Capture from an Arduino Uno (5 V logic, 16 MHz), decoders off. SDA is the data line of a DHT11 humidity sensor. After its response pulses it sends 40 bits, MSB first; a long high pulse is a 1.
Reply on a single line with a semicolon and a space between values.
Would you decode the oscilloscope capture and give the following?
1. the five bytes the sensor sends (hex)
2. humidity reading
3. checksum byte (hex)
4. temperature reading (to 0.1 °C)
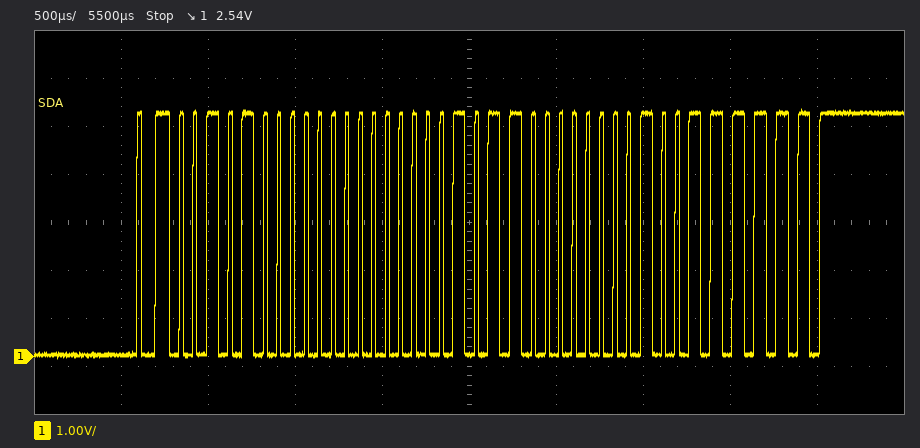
28 00 16 01 3F; 40 %; 0x3F; 22.1 °C
